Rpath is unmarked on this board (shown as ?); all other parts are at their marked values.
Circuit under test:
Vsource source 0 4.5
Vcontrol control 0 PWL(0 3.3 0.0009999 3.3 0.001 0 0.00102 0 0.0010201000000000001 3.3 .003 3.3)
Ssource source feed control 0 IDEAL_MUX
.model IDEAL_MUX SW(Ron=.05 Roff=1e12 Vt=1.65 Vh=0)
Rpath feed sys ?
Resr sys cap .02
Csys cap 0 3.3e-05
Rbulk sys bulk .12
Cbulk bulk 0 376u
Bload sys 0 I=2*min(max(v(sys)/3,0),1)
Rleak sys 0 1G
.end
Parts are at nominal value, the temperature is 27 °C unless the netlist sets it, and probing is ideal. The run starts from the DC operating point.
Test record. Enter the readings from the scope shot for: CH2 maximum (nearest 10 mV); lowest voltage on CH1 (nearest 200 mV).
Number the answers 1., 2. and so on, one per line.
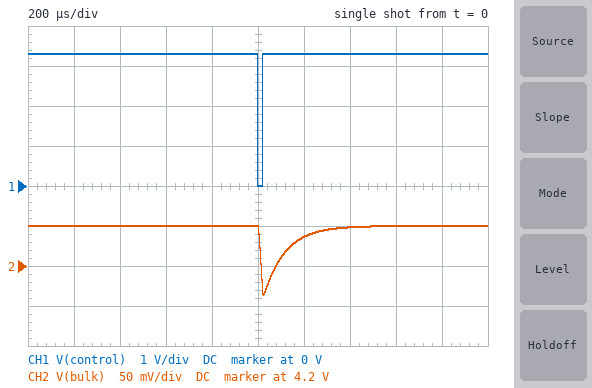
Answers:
1. 4.25 V
2. 0 V
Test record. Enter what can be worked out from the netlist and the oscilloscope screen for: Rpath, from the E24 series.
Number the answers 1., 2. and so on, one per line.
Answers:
1. 0.075 Ω
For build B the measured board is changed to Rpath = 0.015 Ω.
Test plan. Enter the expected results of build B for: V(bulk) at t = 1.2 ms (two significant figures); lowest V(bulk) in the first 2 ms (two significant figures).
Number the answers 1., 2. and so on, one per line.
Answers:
1. 4.4 V
2. 4.3 V
